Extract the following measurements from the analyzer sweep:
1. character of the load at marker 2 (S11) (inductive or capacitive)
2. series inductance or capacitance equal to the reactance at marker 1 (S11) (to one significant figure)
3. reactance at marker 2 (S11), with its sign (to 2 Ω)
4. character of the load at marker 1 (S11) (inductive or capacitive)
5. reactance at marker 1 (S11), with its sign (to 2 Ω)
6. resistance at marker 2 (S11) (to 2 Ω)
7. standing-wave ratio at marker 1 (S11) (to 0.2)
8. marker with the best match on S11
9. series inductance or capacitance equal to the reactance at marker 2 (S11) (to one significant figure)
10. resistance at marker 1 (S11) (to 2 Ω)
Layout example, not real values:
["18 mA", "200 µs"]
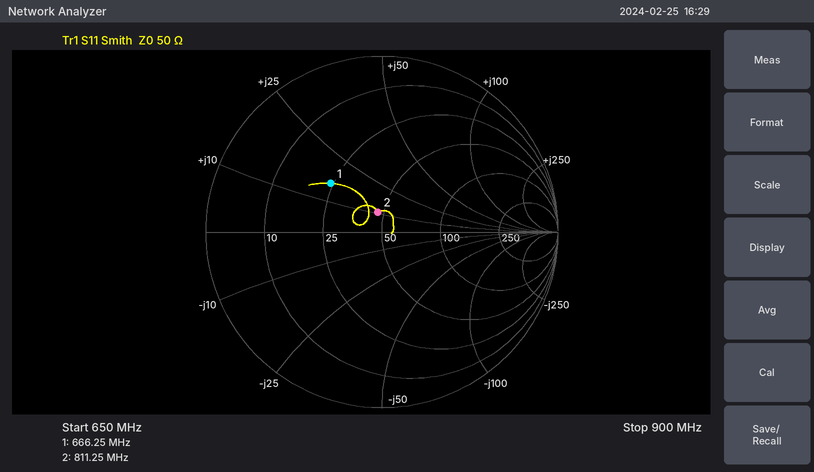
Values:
["inductive", "4 nH", "+10 Ω", "inductive", "+16 Ω", "46 Ω", "2.4", "marker 2", "2 nH", "24 Ω"]
